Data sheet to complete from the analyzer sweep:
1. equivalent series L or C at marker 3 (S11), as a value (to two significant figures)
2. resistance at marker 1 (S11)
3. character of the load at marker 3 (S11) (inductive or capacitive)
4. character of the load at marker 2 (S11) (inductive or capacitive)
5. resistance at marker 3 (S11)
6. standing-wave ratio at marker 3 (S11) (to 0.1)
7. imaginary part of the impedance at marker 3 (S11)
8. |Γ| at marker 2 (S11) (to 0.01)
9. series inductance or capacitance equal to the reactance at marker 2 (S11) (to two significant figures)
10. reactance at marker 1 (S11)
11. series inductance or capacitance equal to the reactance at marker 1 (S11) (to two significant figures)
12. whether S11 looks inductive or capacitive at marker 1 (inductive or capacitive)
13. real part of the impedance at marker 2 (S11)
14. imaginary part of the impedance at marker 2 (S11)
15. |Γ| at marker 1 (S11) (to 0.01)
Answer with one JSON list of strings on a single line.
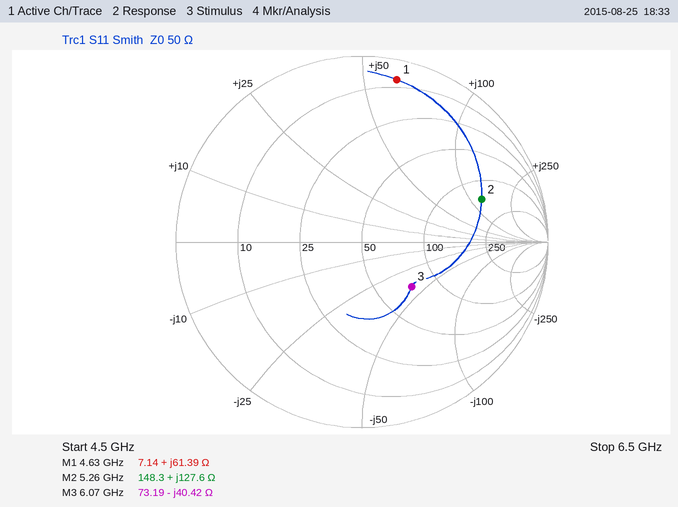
["650 fF", "7.14 Ω", "capacitive", "inductive", "73.19 Ω", "2.1", "-40.42 Ω", "0.68", "3.9 nH", "+61.39 Ω", "2.1 nH", "inductive", "148.3 Ω", "+127.6 Ω", "0.89"]
